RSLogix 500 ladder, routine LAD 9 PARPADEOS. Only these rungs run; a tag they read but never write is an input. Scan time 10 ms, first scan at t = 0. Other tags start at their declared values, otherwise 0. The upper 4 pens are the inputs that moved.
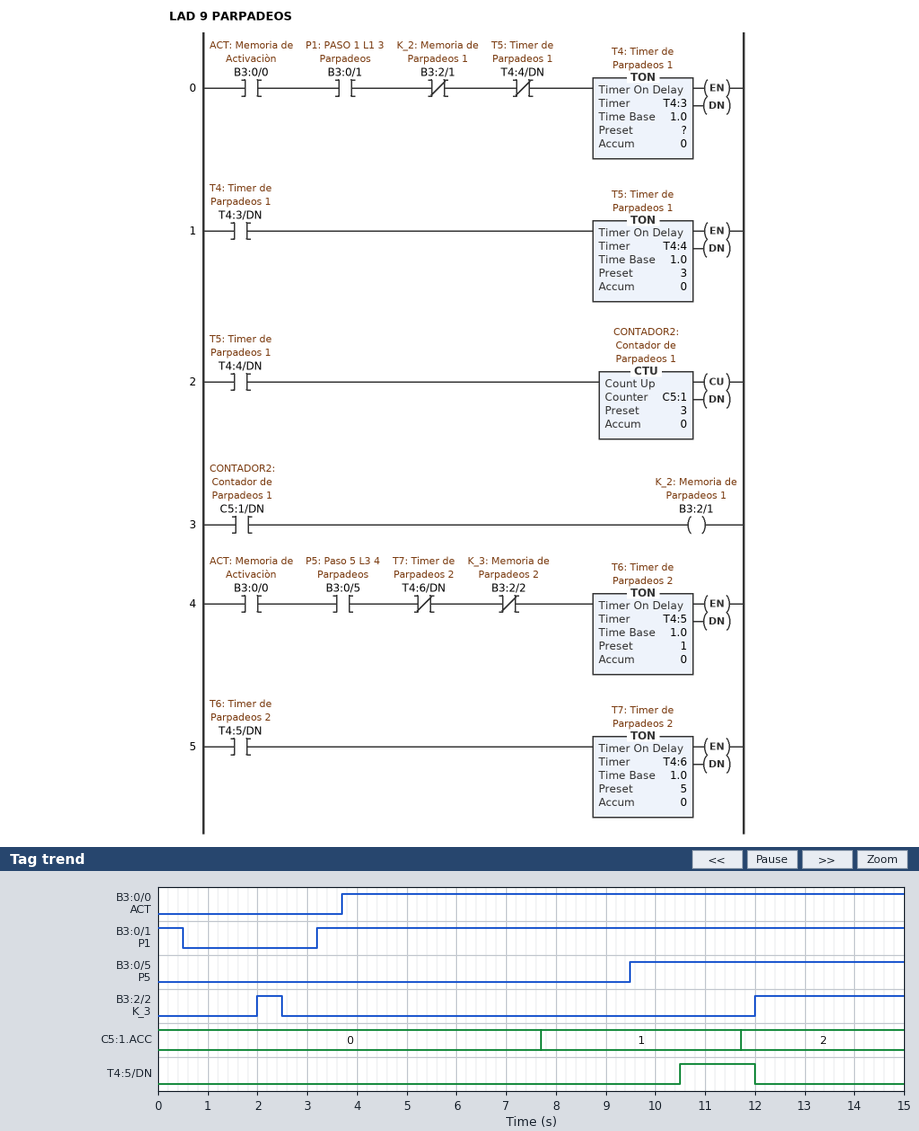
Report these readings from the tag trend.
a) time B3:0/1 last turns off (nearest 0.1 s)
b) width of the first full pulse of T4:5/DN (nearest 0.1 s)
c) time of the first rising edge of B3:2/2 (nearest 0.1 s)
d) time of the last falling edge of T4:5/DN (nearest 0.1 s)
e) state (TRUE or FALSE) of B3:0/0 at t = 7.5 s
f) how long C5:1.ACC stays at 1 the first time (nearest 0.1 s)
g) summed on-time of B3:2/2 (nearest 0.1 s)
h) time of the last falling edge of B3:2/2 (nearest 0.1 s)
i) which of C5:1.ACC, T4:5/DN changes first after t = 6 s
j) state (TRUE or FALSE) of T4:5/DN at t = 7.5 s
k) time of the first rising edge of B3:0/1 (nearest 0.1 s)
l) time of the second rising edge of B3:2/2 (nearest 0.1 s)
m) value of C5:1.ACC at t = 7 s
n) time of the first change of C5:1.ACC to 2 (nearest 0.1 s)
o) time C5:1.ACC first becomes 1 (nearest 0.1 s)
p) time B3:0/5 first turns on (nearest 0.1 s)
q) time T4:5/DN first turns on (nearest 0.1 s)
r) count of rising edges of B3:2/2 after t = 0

0.5 s
1.5 s
2.0 s
12.0 s
TRUE
4.0 s
3.5 s
2.5 s
C5:1.ACC
FALSE
3.2 s
12.0 s
0
11.7 s
7.7 s
9.5 s
10.5 s
2
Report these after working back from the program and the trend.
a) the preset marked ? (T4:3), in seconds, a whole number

1 s
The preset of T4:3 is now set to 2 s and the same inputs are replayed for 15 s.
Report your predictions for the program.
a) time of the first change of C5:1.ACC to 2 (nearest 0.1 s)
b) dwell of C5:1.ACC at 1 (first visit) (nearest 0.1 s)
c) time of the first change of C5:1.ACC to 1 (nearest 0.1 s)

13.7 s
5.0 s
8.7 s
